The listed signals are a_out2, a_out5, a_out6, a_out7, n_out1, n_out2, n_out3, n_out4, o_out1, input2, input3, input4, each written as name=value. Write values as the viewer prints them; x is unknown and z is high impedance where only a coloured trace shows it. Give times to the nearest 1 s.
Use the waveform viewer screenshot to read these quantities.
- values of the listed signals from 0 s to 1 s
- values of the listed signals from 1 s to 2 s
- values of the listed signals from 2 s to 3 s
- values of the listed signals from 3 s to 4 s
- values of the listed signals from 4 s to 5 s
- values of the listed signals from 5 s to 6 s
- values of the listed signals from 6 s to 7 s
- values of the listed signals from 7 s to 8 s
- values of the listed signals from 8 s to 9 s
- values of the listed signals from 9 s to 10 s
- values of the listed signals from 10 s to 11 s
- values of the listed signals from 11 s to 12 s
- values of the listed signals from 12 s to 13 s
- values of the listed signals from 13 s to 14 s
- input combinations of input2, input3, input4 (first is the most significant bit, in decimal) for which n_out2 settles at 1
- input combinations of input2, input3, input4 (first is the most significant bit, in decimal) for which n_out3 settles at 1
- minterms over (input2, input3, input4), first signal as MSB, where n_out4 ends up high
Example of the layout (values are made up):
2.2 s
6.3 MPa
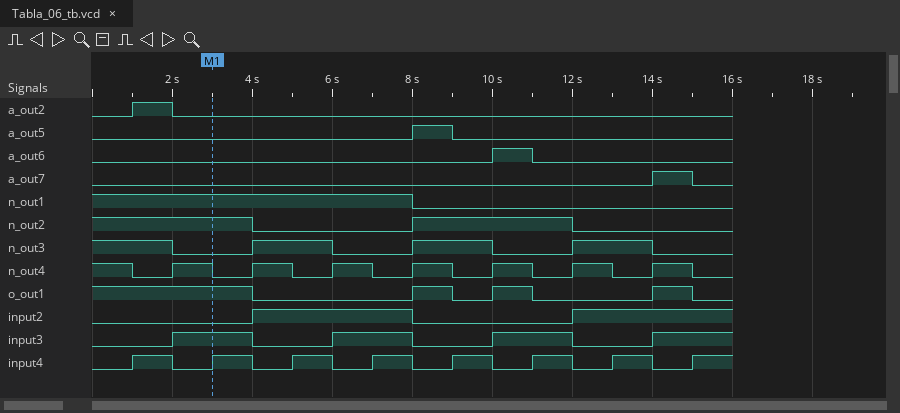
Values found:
a_out2=0, a_out5=0, a_out6=0, a_out7=0, n_out1=1, n_out2=1, n_out3=1, n_out4=1, o_out1=1, input2=0, input3=0, input4=0
a_out2=1, a_out5=0, a_out6=0, a_out7=0, n_out1=1, n_out2=1, n_out3=1, n_out4=0, o_out1=1, input2=0, input3=0, input4=1
a_out2=0, a_out5=0, a_out6=0, a_out7=0, n_out1=1, n_out2=1, n_out3=0, n_out4=1, o_out1=1, input2=0, input3=1, input4=0
a_out2=0, a_out5=0, a_out6=0, a_out7=0, n_out1=1, n_out2=1, n_out3=0, n_out4=0, o_out1=1, input2=0, input3=1, input4=1
a_out2=0, a_out5=0, a_out6=0, a_out7=0, n_out1=1, n_out2=0, n_out3=1, n_out4=1, o_out1=0, input2=1, input3=0, input4=0
a_out2=0, a_out5=0, a_out6=0, a_out7=0, n_out1=1, n_out2=0, n_out3=1, n_out4=0, o_out1=0, input2=1, input3=0, input4=1
a_out2=0, a_out5=0, a_out6=0, a_out7=0, n_out1=1, n_out2=0, n_out3=0, n_out4=1, o_out1=0, input2=1, input3=1, input4=0
a_out2=0, a_out5=0, a_out6=0, a_out7=0, n_out1=1, n_out2=0, n_out3=0, n_out4=0, o_out1=0, input2=1, input3=1, input4=1
a_out2=0, a_out5=1, a_out6=0, a_out7=0, n_out1=0, n_out2=1, n_out3=1, n_out4=1, o_out1=1, input2=0, input3=0, input4=0
a_out2=0, a_out5=0, a_out6=0, a_out7=0, n_out1=0, n_out2=1, n_out3=1, n_out4=0, o_out1=0, input2=0, input3=0, input4=1
a_out2=0, a_out5=0, a_out6=1, a_out7=0, n_out1=0, n_out2=1, n_out3=0, n_out4=1, o_out1=1, input2=0, input3=1, input4=0
a_out2=0, a_out5=0, a_out6=0, a_out7=0, n_out1=0, n_out2=1, n_out3=0, n_out4=0, o_out1=0, input2=0, input3=1, input4=1
a_out2=0, a_out5=0, a_out6=0, a_out7=0, n_out1=0, n_out2=0, n_out3=1, n_out4=1, o_out1=0, input2=1, input3=0, input4=0
a_out2=0, a_out5=0, a_out6=0, a_out7=0, n_out1=0, n_out2=0, n_out3=1, n_out4=0, o_out1=0, input2=1, input3=0, input4=1
0, 1, 2, 3
0, 1, 4, 5
0, 2, 4, 6
